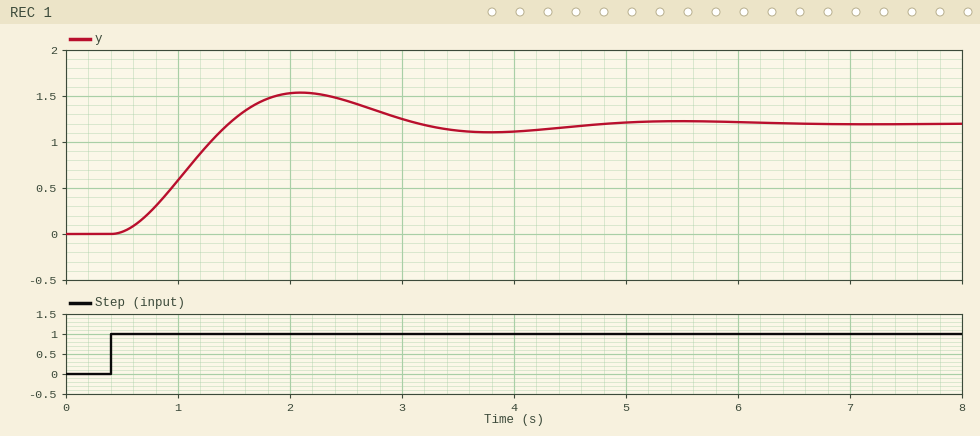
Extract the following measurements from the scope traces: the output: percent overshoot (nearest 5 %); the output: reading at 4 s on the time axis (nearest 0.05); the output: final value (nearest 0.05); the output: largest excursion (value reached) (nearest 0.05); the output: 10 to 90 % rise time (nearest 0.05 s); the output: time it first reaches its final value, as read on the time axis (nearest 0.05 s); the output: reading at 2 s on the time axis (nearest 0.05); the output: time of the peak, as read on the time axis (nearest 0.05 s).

30 %
1.10
1.20
1.55
0.70 s
1.45 s
1.55
2.10 s
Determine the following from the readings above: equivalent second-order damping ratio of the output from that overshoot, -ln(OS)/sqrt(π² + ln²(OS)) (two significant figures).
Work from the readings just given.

0.36
